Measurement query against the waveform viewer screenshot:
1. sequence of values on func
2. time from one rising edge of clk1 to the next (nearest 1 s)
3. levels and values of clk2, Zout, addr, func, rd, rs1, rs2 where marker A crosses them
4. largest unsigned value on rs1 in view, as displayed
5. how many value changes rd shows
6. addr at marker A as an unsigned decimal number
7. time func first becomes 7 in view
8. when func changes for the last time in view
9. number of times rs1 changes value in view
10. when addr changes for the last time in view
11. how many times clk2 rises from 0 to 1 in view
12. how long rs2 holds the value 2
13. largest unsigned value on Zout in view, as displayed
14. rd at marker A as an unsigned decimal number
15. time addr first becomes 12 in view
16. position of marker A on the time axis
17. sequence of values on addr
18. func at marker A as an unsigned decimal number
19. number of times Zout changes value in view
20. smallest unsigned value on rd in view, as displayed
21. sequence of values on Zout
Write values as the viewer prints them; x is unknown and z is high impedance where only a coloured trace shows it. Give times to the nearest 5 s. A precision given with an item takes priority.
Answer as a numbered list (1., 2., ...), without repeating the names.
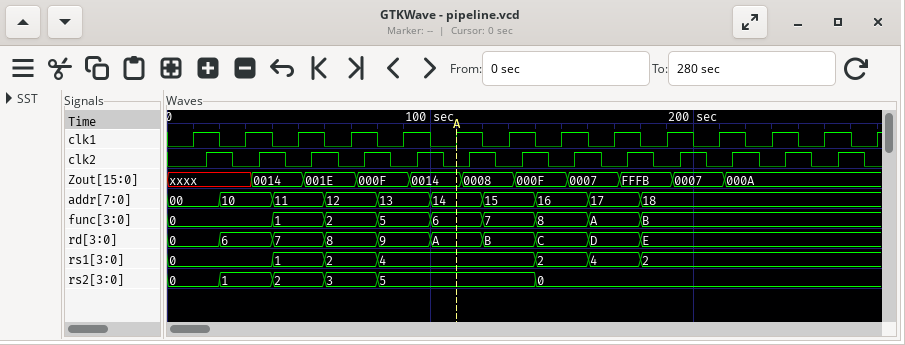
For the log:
1. 0, 1, 2, 5, 6, 7, 8, A, B
2. 20 s
3. clk2=0, Zout=0014, addr=14, func=6, rd=A, rs1=4, rs2=5
4. 4
5. 9
6. 20
7. 120 s
8. 180 s
9. 6
10. 180 s
11. 13
12. 20 s
13. FFFB
14. 10
15. 60 s
16. 110 s
17. 00, 10, 11, 12, 13, 14, 15, 16, 17, 18
18. 6
19. 10
20. 0
21. xxxx, 0014, 001E, 000F, 0014, 0008, 000F, 0007, FFFB, 0007, 000A
